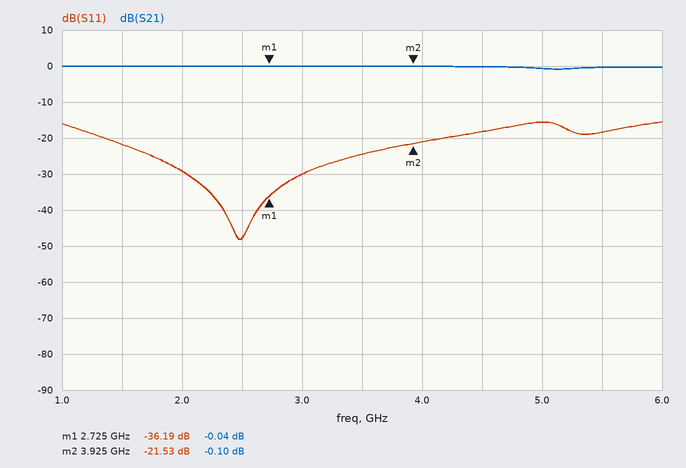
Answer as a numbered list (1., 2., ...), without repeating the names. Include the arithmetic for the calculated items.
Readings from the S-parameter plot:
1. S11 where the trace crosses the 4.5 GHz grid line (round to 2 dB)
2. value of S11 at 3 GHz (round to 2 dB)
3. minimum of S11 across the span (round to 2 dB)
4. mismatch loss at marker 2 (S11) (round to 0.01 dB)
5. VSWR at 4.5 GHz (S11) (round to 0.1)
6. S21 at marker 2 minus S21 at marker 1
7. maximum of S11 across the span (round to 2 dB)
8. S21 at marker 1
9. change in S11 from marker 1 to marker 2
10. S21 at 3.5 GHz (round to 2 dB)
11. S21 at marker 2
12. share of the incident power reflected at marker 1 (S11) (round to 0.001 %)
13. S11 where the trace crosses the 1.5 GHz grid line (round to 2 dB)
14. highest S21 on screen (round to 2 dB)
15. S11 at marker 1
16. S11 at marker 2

1. -18 dB
2. -30 dB
3. -48 dB
4. −10 log10(1 − 10^(-21.53/10)) ≈ 0.03 dB
5. |Γ| = 10^(-18/20) = 0.1259; VSWR = (1 + 0.1259)/(1 − 0.1259) ≈ 1.3
6. -0.1 − (-0.04) = -0.06 dB
7. -16 dB
8. -0.04 dB
9. -21.53 − (-36.19) = 14.66 dB
10. 0 dB
11. -0.10 dB
12. 10^(-36.19/10) ≈ 0.024 %
13. -22 dB
14. 0 dB
15. -36.19 dB
16. -21.53 dB
